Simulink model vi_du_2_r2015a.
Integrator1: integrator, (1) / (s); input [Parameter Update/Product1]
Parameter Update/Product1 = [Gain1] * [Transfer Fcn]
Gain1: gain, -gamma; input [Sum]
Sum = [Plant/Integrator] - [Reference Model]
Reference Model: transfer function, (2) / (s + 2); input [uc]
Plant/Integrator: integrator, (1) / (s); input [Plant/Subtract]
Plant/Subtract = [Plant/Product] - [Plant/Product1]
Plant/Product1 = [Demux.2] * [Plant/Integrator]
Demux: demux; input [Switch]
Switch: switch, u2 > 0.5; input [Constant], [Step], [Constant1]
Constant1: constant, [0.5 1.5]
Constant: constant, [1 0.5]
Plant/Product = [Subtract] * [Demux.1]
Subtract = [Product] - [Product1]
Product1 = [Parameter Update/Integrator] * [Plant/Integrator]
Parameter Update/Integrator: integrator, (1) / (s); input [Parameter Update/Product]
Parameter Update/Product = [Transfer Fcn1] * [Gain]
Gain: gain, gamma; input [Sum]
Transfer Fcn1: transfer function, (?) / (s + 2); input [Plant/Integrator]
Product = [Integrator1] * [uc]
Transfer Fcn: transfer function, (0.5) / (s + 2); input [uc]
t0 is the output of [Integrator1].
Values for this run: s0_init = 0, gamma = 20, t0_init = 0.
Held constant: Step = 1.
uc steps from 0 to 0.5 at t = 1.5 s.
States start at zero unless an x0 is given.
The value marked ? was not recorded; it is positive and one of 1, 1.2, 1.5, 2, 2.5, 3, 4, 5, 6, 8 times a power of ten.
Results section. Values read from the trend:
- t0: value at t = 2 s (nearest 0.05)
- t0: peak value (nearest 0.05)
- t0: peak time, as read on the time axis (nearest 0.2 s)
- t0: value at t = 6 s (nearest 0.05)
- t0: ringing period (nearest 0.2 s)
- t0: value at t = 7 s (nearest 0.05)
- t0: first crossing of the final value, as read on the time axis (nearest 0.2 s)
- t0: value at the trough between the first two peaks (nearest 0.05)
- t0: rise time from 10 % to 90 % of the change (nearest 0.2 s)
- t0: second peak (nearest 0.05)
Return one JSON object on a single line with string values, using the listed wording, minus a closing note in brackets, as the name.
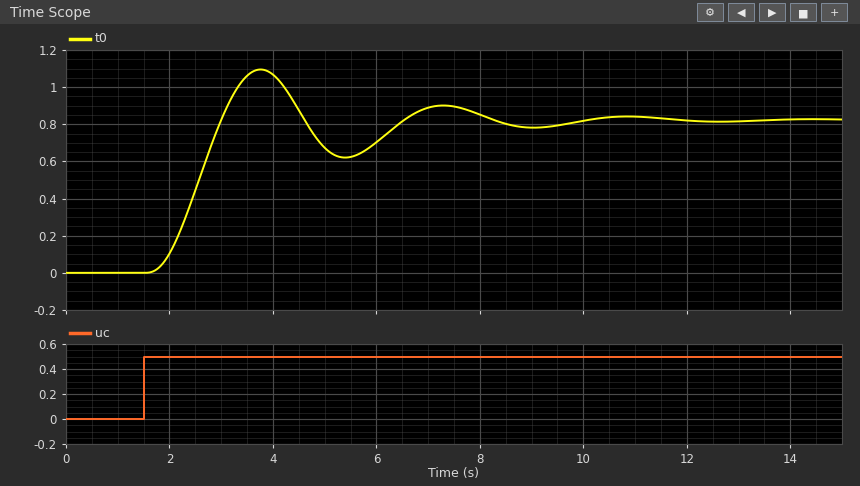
{"t0: value at t = 2 s": "0.10", "t0: peak value": "1.10", "t0: peak time, as read on the time axis": "3.8 s", "t0: value at t = 6 s": "0.70", "t0: ringing period": "3.6 s", "t0: value at t = 7 s": "0.90", "t0: first crossing of the final value, as read on the time axis": "3.0 s", "t0: value at the trough between the first two peaks": "0.60", "t0: rise time from 10 % to 90 % of the change": "1.0 s", "t0: second peak": "0.90"}
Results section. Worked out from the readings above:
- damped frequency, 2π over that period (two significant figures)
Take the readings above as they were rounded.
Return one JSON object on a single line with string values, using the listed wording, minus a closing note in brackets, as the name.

{"damped frequency, 2π over that period": "1.7 rad/s"}
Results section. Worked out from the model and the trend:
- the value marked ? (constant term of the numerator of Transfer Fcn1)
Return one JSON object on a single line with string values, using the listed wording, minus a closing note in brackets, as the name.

{"the value marked ?": "0.8"}
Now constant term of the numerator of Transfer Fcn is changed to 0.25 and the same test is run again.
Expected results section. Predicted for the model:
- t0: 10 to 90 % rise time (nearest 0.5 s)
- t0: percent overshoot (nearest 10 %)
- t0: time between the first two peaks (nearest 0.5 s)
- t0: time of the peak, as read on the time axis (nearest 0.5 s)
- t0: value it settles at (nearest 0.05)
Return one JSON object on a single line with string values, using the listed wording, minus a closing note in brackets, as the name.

{"t0: 10 to 90 % rise time": "1.5 s", "t0: percent overshoot": "20 %", "t0: time between the first two peaks": "4.0 s", "t0: time of the peak, as read on the time axis": "4.5 s", "t0: value it settles at": "0.70"}
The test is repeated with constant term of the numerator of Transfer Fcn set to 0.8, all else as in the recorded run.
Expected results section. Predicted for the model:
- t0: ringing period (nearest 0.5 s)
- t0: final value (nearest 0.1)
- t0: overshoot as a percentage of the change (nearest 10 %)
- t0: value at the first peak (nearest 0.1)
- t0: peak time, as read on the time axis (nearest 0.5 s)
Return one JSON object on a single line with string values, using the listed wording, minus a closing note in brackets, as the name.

{"t0: ringing period": "3.0 s", "t0: final value": "0.9", "t0: overshoot as a percentage of the change": "50 %", "t0: value at the first peak": "1.3", "t0: peak time, as read on the time axis": "3.5 s"}
